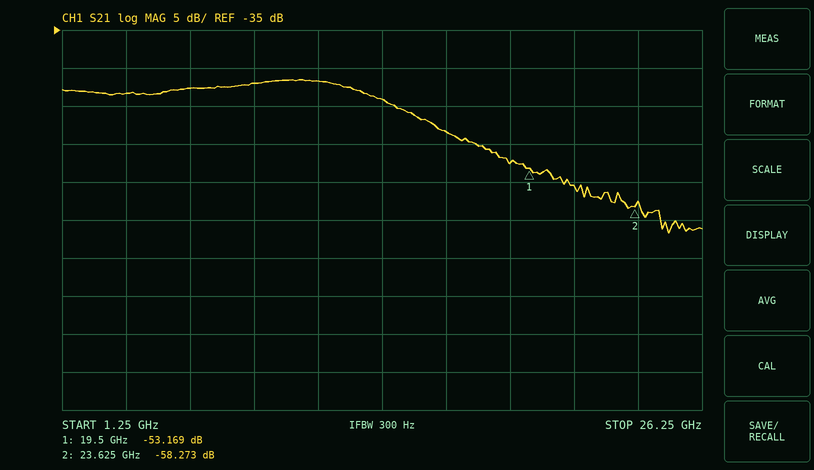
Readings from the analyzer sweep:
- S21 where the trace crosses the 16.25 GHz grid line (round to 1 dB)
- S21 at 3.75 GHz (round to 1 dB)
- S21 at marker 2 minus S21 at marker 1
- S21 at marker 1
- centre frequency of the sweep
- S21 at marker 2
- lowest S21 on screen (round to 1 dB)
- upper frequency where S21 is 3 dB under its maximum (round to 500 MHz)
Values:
-48 dB
-43 dB
-5.104 dB
-53.169 dB
13.75 GHz
-58.273 dB
-62 dB
14.0 GHz
